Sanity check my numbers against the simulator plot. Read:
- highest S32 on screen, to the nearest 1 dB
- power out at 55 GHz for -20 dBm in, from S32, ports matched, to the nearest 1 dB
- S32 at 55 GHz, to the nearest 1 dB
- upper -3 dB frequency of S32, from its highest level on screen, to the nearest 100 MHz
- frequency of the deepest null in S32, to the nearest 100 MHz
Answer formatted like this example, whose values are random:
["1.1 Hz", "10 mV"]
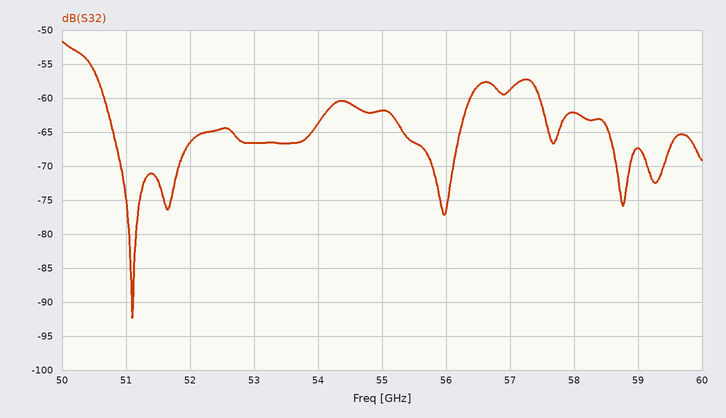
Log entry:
["-52 dB", "-82 dBm", "-62 dB", "50.4 GHz", "51.1 GHz"]
